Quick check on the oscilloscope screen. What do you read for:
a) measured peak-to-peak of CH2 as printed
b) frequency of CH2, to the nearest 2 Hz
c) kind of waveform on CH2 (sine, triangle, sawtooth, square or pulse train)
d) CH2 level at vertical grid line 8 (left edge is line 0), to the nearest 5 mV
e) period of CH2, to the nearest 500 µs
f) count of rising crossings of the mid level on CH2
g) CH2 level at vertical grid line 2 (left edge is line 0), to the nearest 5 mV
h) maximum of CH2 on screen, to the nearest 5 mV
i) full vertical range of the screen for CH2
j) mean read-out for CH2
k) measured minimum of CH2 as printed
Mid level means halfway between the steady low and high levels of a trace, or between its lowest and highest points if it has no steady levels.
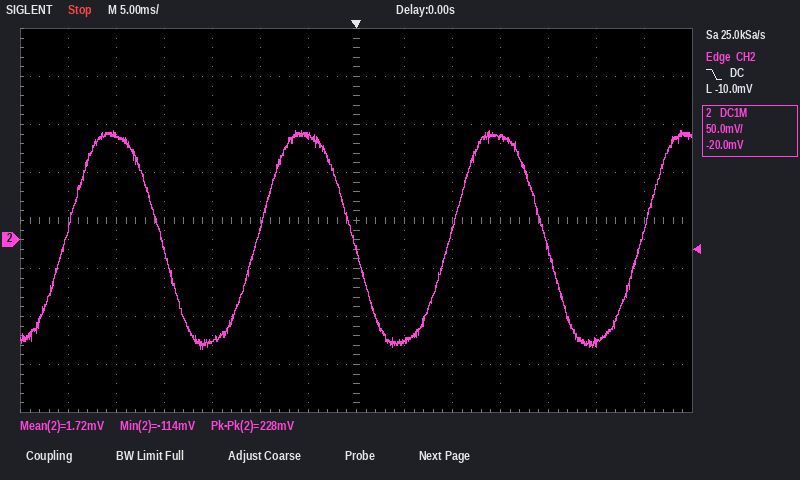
228 mV
50 Hz
sine
-105 mV
20.0 ms
4
110 mV
115 mV
400 mV
1.72 mV
-114 mV
